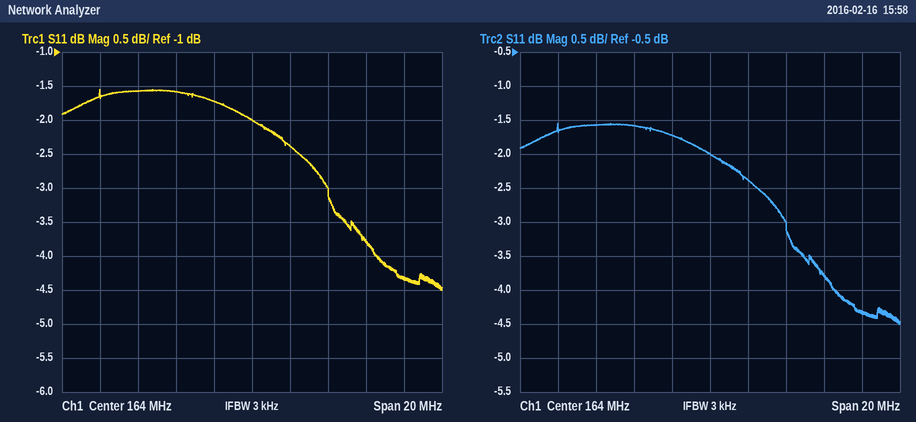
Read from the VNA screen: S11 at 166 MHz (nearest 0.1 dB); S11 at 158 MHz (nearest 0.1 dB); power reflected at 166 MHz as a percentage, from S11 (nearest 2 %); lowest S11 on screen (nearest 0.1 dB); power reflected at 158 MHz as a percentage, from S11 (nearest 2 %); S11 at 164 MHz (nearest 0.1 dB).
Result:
-2.4 dB
-1.6 dB
58 %
-4.5 dB
70 %
-2.0 dB
